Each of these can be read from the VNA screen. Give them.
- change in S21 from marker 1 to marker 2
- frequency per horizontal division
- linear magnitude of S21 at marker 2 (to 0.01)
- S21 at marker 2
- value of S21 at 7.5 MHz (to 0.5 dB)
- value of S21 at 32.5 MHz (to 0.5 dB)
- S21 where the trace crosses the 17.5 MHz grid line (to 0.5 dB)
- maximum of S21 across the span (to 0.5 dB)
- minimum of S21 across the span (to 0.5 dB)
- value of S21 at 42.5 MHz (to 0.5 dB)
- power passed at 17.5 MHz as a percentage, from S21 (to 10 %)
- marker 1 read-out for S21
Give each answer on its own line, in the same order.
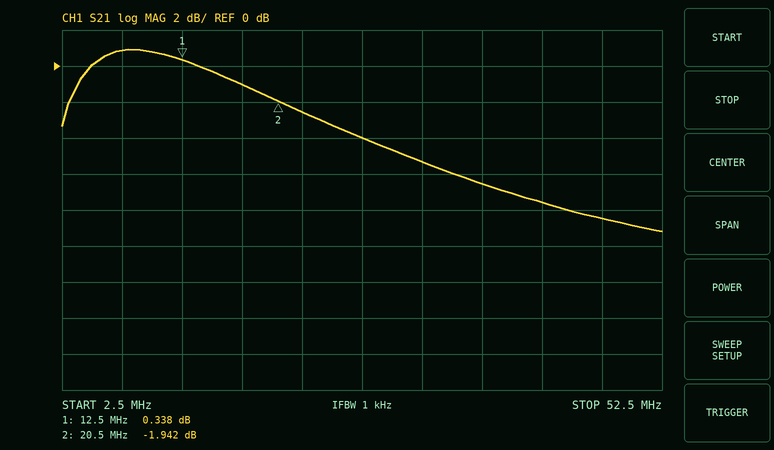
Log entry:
-2.280 dB
5 MHz
0.80
-1.942 dB
1.0 dB
-5.5 dB
-1.0 dB
1.0 dB
-9.0 dB
-7.5 dB
80 %
0.338 dB
